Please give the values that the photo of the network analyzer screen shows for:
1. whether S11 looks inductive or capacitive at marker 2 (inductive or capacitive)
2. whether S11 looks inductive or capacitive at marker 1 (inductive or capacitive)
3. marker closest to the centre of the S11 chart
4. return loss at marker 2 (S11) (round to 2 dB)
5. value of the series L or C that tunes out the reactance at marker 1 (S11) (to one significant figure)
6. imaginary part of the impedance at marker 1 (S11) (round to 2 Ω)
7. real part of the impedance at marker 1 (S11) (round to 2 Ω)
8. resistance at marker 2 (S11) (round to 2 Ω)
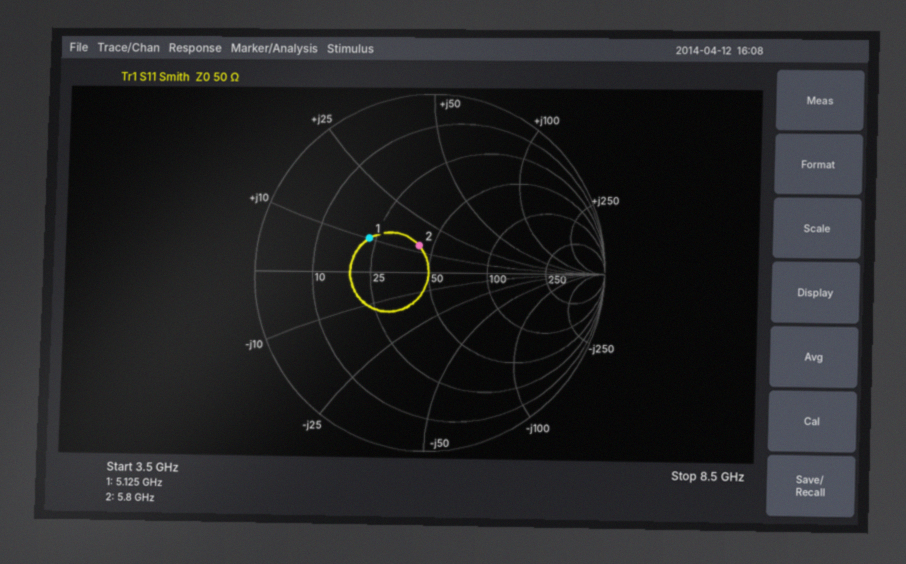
inductive
inductive
marker 2
16 dB
3 pF
+10 Ω
22 Ω
42 Ω
